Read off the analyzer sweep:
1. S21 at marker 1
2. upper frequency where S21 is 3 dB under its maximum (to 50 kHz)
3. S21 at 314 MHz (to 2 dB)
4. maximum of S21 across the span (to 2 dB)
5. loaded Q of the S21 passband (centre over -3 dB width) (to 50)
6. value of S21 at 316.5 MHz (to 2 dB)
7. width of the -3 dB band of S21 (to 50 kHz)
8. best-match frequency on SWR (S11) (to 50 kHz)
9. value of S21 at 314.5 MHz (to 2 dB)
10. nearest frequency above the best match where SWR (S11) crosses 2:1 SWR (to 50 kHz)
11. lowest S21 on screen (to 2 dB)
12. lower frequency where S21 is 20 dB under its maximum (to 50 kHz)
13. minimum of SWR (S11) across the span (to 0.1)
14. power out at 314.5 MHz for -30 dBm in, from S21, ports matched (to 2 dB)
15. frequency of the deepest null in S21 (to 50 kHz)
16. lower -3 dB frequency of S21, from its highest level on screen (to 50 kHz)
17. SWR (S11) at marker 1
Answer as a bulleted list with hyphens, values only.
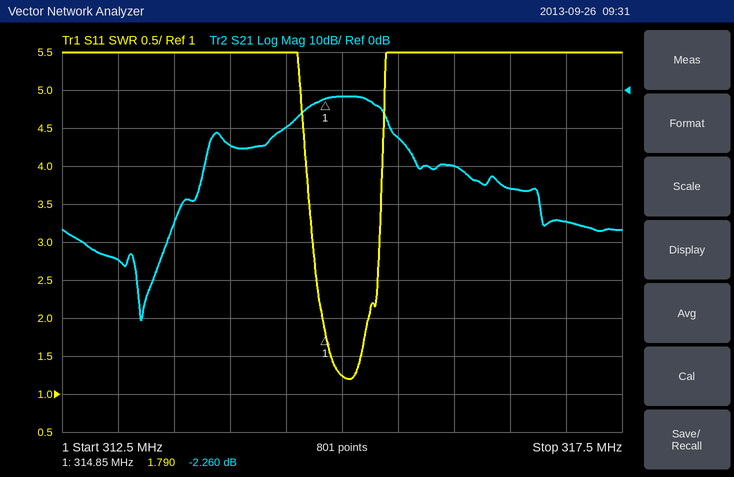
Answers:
- -2.260 dB
- 315.35 MHz
- -14 dB
- -2 dB
- 500
- -26 dB
- 650 kHz
- 315.05 MHz
- -10 dB
- 315.25 MHz
- -60 dB
- 313.75 MHz
- 1.2
- -40 dBm
- 313.20 MHz
- 314.70 MHz
- 1.790
